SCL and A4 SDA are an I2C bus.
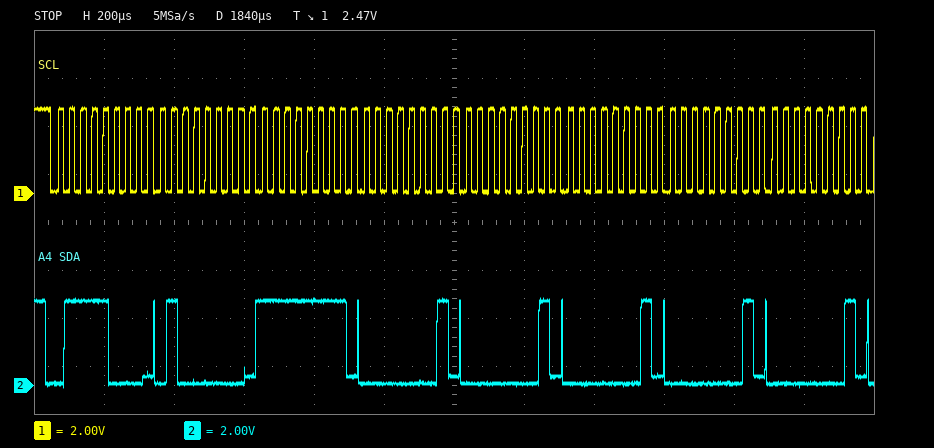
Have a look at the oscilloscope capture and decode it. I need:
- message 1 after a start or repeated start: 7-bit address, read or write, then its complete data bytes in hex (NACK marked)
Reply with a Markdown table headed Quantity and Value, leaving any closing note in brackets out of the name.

| Quantity | Value |
|---|---|
| message 1 after a start or repeated start: 7-bit address, read or write, then its complete data bytes in hex | 0x3C write: 40 FF 01 01 01 01 01 |
